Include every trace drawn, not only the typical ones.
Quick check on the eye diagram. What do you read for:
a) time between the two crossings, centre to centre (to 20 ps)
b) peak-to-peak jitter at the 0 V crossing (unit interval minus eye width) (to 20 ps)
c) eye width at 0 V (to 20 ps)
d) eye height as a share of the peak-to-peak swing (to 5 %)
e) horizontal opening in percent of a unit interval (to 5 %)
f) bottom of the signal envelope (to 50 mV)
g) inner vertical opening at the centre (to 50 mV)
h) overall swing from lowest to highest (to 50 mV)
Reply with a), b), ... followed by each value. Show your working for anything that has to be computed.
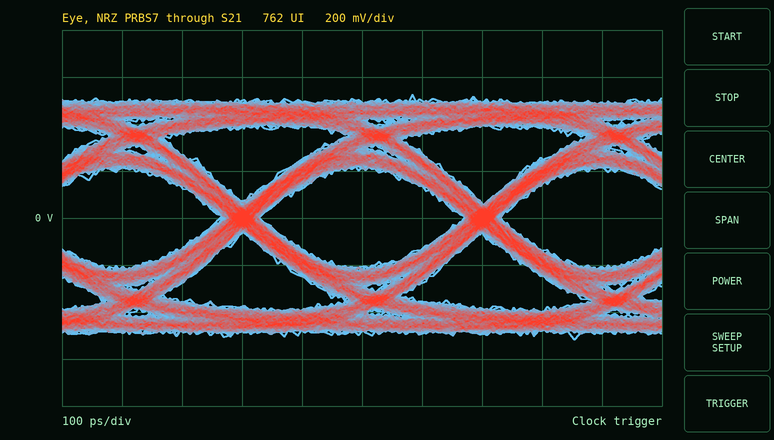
a) 400 ps
b) 60 ps
c) 340 ps
d) 400 mV / 1.05 V ≈ 38.1 %, so 40 % to the nearest 5 %
e) 340 ps / 400 ps ≈ 85 %
f) -500 mV
g) 400 mV
h) 1.05 V
